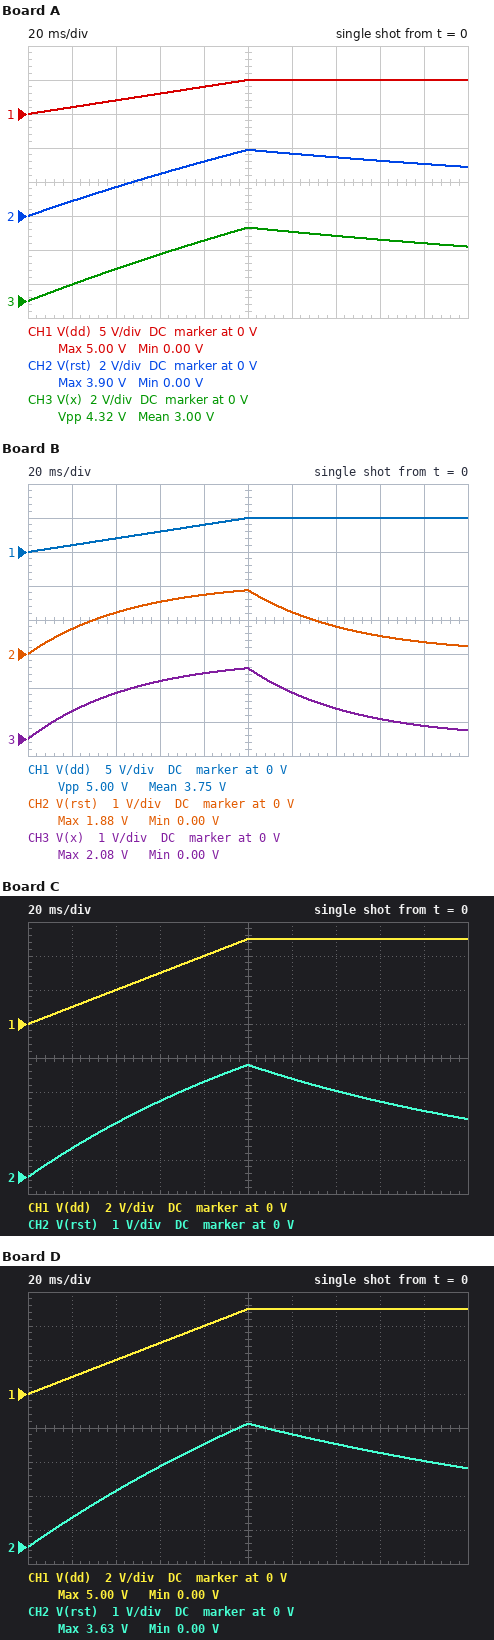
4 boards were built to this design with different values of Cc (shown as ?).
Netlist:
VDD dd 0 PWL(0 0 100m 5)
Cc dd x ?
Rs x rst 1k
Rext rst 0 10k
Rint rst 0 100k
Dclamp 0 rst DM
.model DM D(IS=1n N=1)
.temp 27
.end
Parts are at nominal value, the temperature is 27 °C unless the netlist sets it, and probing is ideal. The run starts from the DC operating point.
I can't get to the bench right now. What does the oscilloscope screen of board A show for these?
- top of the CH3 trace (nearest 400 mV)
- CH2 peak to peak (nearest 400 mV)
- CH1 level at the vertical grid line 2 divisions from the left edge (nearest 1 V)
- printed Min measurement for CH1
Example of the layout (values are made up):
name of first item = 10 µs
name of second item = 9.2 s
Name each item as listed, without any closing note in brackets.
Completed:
top of the CH3 trace = 4.4 V
CH2 peak to peak = 4.0 V
CH1 level at the vertical grid line 2 divisions from the left edge = 2 V
printed Min measurement for CH1 = 0.00 V
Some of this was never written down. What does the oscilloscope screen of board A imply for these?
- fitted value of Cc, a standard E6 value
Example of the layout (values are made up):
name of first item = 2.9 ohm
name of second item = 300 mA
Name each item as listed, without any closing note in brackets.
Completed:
fitted value of Cc, a standard E6 value = 33 µF
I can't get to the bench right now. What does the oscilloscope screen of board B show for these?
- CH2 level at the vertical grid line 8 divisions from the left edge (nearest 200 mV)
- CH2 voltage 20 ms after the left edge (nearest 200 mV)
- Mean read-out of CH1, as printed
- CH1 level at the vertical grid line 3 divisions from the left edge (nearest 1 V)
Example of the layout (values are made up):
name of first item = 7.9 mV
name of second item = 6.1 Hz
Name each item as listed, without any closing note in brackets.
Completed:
CH2 level at the vertical grid line 8 divisions from the left edge = 600 mV
CH2 voltage 20 ms after the left edge = 800 mV
Mean read-out of CH1, as printed = 3.75 V
CH1 level at the vertical grid line 3 divisions from the left edge = 3 V
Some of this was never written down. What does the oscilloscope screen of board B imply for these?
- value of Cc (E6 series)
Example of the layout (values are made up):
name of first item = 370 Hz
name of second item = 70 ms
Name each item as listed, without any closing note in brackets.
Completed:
value of Cc = 4.7 µF
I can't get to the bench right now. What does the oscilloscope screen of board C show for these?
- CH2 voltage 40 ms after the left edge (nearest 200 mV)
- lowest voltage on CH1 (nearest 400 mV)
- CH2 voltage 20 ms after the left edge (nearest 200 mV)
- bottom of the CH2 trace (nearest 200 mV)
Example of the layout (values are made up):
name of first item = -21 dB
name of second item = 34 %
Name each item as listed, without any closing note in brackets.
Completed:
CH2 voltage 40 ms after the left edge = 1.6 V
lowest voltage on CH1 = 0 V
CH2 voltage 20 ms after the left edge = 800 mV
bottom of the CH2 trace = 0 V
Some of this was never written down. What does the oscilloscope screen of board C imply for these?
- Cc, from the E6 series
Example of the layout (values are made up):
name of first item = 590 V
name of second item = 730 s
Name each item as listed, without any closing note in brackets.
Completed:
Cc, from the E6 series = 15 µF
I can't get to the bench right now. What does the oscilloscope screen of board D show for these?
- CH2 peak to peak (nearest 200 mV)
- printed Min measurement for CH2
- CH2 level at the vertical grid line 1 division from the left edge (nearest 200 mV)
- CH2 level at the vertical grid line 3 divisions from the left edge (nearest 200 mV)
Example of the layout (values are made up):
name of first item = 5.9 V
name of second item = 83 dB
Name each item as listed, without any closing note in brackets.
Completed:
CH2 peak to peak = 3.6 V
printed Min measurement for CH2 = 0.00 V
CH2 level at the vertical grid line 1 division from the left edge = 800 mV
CH2 level at the vertical grid line 3 divisions from the left edge = 2.4 V
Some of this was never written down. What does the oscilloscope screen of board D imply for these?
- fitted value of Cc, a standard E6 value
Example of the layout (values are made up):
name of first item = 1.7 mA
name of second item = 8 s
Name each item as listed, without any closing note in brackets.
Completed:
fitted value of Cc, a standard E6 value = 22 µF
